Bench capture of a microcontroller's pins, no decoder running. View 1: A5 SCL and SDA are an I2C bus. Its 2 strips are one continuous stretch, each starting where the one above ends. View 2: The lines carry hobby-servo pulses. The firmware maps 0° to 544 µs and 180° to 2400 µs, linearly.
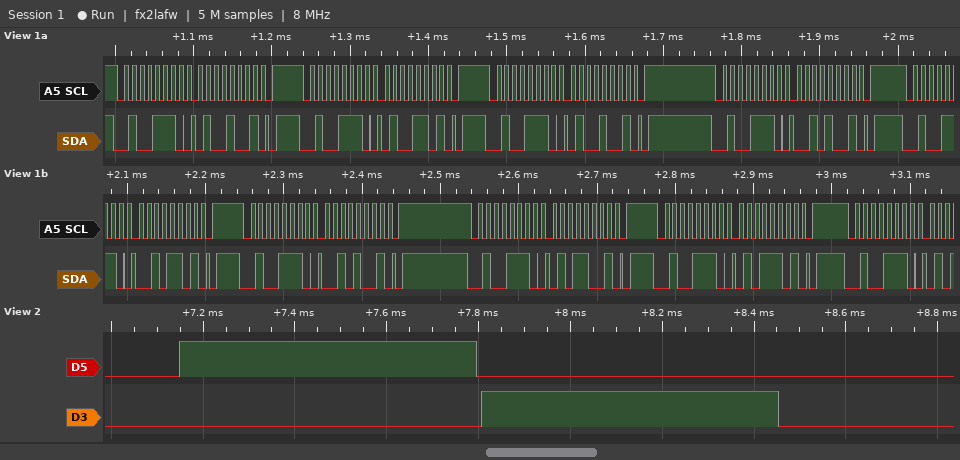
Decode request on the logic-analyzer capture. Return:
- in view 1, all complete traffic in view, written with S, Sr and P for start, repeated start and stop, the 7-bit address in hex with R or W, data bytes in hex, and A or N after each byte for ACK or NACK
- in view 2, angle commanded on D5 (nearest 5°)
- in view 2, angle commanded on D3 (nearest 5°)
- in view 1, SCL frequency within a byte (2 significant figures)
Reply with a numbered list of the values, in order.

1. S 27W A 49 A P S 27W A 4D A P S 27W A 49 A P S 27W A 29 A P S 27W A 2D A P S 27W A 29 A P S 27W A 59 A P S 27W A 5D A P S 27W A
2. 10°
3. 10°
4. 100 kHz
